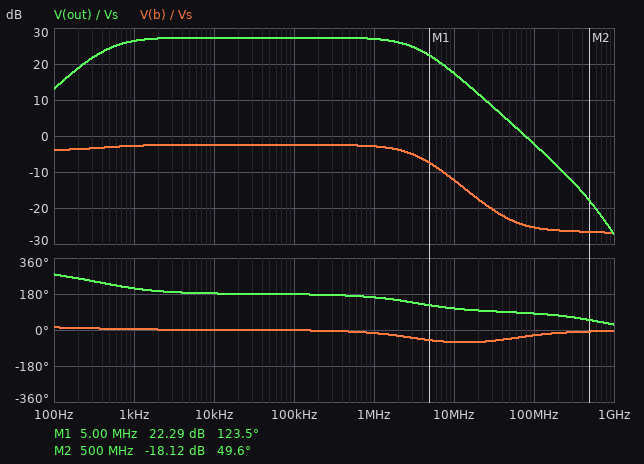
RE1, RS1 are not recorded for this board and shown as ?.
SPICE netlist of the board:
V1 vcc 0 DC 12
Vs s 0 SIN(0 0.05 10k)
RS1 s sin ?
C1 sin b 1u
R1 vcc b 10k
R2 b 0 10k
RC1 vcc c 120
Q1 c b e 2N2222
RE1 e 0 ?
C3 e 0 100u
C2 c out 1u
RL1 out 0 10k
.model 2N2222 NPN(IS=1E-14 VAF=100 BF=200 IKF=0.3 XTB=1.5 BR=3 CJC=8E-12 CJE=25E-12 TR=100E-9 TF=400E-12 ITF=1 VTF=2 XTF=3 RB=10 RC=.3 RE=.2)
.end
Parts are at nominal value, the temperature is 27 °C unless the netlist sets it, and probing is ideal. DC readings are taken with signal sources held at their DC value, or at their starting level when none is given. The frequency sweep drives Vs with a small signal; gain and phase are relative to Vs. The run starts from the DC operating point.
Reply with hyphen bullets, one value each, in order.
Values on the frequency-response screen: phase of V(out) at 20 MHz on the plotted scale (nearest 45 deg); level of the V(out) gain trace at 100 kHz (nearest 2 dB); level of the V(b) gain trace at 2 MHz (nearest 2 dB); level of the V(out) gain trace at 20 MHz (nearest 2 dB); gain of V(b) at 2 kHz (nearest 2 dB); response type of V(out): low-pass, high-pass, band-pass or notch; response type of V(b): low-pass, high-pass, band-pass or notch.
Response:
- 90 deg
- 28 dB
- -4 dB
- 12 dB
- -2 dB
- band-pass
- low-pass
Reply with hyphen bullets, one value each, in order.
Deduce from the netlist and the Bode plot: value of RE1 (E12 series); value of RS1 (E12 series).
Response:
- 680 Ω
- 220 Ω
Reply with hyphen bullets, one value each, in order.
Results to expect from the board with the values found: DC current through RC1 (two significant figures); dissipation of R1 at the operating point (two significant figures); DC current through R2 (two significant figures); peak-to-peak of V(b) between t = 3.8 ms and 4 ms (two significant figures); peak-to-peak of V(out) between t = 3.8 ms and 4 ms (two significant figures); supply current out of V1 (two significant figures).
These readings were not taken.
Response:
- 7.5 mA
- 3.8 mW
- 580 µA
- 78 mV
- 2.0 V
- 8.1 mA
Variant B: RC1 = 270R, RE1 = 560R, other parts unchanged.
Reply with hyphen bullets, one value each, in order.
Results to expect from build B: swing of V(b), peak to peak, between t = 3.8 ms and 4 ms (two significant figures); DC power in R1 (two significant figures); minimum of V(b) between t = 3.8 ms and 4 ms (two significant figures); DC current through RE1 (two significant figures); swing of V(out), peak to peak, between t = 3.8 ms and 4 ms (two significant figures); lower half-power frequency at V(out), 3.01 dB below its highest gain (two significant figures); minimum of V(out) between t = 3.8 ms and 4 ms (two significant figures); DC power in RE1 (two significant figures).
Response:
- 75 mV
- 3.9 mW
- 5.7 V
- 9.0 mA
- 4.9 V
- 550 Hz
- -2.9 V
- 46 mW
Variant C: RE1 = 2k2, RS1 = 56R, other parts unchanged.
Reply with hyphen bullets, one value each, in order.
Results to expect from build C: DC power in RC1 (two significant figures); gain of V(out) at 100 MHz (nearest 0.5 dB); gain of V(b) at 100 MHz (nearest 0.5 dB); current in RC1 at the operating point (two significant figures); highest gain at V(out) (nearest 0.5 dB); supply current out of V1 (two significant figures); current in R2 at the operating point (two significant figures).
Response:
- 680 µW
- 6.0 dB
- -12.0 dB
- 2.4 mA
- 20.0 dB
- 3.0 mA
- 590 µA
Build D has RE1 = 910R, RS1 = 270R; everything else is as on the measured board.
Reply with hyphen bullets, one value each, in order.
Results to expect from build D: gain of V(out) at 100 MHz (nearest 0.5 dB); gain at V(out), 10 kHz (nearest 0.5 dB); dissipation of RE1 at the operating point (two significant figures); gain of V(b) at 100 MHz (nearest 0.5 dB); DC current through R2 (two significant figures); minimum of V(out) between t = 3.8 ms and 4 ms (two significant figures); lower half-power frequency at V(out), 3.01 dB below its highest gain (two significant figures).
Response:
- -4.5 dB
- 25.0 dB
- 29 mW
- -26.5 dB
- 590 µA
- -940 mV
- 380 Hz
